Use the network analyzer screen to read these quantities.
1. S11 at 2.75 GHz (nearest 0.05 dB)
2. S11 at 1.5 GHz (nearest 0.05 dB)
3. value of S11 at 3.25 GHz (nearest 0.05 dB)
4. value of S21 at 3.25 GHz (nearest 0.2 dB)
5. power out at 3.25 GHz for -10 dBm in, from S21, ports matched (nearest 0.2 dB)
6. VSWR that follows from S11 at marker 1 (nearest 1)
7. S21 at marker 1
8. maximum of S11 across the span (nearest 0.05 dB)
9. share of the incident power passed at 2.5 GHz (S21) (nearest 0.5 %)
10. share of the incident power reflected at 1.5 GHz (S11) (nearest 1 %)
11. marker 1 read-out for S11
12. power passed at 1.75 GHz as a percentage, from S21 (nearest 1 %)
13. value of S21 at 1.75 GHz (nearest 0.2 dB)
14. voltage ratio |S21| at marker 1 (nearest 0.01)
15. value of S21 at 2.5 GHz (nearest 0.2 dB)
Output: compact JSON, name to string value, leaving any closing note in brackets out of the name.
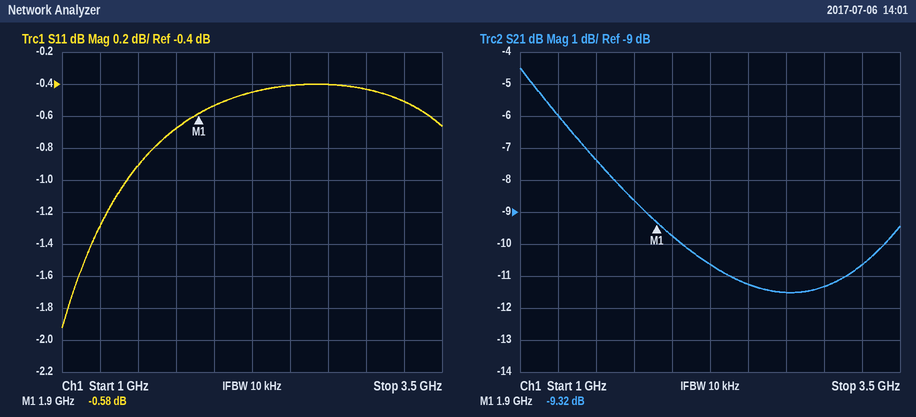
{"S11 at 2.75 GHz": "-0.40 dB", "S11 at 1.5 GHz": "-0.90 dB", "value of S11 at 3.25 GHz": "-0.50 dB", "value of S21 at 3.25 GHz": "-10.6 dB", "power out at 3.25 GHz for -10 dBm in, from S21, ports matched": "-20.6 dBm", "VSWR that follows from S11 at marker 1": "30", "S21 at marker 1": "-9.32 dB", "maximum of S11 across the span": "-0.40 dB", "share of the incident power passed at 2.5 GHz (S21)": "7.5 %", "share of the incident power reflected at 1.5 GHz (S11)": "81 %", "marker 1 read-out for S11": "-0.58 dB", "power passed at 1.75 GHz as a percentage, from S21": "14 %", "value of S21 at 1.75 GHz": "-8.6 dB", "voltage ratio |S21| at marker 1": "0.34", "value of S21 at 2.5 GHz": "-11.2 dB"}
